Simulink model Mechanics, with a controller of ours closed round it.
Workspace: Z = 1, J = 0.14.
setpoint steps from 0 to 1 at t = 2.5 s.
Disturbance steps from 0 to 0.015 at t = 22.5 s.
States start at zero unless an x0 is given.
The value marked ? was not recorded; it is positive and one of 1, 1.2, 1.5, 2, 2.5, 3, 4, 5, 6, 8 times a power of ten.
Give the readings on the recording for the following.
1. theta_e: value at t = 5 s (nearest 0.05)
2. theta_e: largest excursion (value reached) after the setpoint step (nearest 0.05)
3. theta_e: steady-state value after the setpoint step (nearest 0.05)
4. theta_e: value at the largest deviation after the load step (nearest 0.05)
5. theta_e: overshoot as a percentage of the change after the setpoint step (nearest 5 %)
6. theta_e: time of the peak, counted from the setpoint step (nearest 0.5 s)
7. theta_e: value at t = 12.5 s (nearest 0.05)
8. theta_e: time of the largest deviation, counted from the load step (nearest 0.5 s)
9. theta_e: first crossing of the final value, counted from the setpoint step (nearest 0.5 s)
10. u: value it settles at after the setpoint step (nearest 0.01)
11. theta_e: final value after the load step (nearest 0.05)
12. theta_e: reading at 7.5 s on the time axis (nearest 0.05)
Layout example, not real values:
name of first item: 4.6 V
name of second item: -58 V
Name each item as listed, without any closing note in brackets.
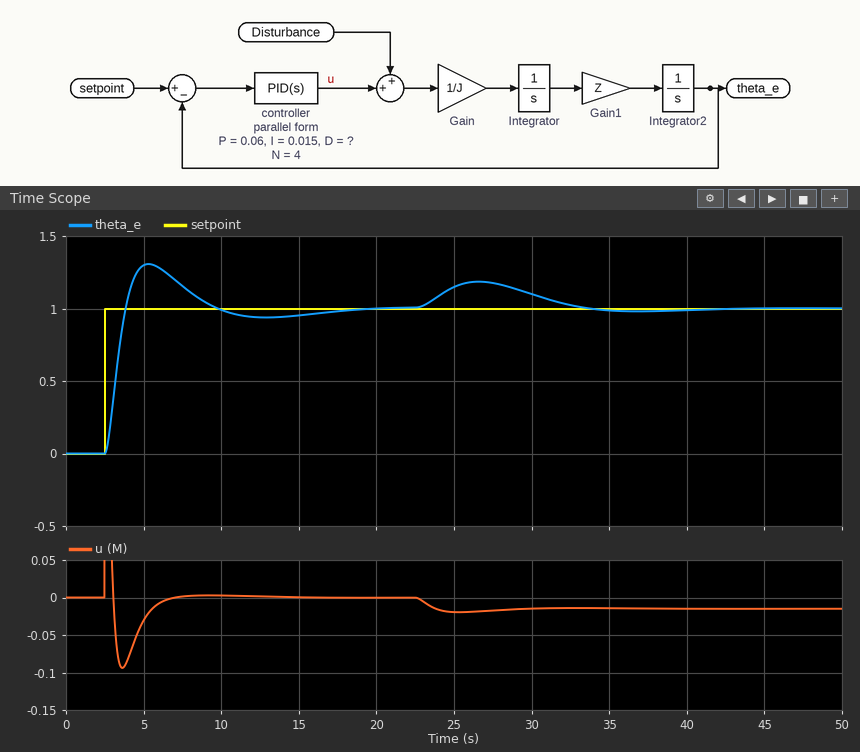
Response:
theta_e: value at t = 5 s: 1.30
theta_e: largest excursion (value reached) after the setpoint step: 1.30
theta_e: steady-state value after the setpoint step: 1.00
theta_e: value at the largest deviation after the load step: 1.20
theta_e: overshoot as a percentage of the change after the setpoint step: 30 %
theta_e: time of the peak, counted from the setpoint step: 3.0 s
theta_e: value at t = 12.5 s: 0.95
theta_e: time of the largest deviation, counted from the load step: 4.0 s
theta_e: first crossing of the final value, counted from the setpoint step: 1.5 s
u: value it settles at after the setpoint step: 0.00
theta_e: final value after the load step: 1.00
theta_e: reading at 7.5 s on the time axis: 1.15
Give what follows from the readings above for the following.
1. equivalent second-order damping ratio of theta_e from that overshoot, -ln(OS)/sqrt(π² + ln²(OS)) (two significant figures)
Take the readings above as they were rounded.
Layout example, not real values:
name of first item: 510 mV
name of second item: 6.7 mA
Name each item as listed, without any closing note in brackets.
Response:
equivalent second-order damping ratio of theta_e from that overshoot, -ln(OS)/sqrt(π² + ln²(OS)): 0.36
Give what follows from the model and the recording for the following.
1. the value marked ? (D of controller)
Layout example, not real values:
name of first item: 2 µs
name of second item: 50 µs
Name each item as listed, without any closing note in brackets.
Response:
the value marked ?: 0.15
